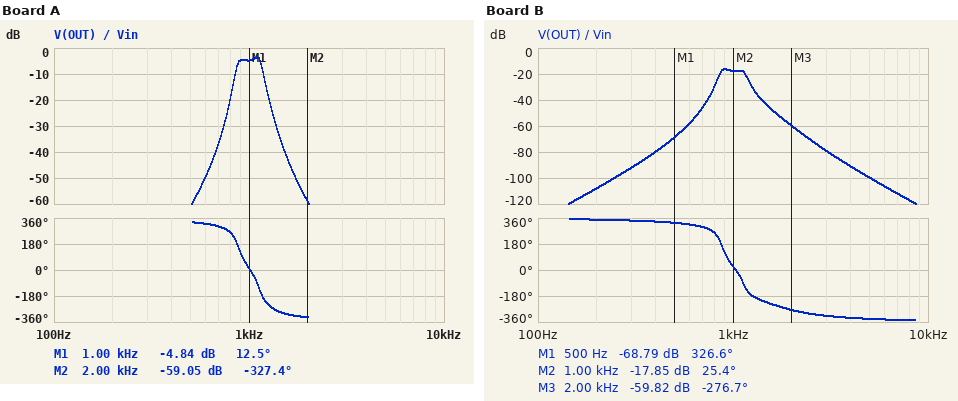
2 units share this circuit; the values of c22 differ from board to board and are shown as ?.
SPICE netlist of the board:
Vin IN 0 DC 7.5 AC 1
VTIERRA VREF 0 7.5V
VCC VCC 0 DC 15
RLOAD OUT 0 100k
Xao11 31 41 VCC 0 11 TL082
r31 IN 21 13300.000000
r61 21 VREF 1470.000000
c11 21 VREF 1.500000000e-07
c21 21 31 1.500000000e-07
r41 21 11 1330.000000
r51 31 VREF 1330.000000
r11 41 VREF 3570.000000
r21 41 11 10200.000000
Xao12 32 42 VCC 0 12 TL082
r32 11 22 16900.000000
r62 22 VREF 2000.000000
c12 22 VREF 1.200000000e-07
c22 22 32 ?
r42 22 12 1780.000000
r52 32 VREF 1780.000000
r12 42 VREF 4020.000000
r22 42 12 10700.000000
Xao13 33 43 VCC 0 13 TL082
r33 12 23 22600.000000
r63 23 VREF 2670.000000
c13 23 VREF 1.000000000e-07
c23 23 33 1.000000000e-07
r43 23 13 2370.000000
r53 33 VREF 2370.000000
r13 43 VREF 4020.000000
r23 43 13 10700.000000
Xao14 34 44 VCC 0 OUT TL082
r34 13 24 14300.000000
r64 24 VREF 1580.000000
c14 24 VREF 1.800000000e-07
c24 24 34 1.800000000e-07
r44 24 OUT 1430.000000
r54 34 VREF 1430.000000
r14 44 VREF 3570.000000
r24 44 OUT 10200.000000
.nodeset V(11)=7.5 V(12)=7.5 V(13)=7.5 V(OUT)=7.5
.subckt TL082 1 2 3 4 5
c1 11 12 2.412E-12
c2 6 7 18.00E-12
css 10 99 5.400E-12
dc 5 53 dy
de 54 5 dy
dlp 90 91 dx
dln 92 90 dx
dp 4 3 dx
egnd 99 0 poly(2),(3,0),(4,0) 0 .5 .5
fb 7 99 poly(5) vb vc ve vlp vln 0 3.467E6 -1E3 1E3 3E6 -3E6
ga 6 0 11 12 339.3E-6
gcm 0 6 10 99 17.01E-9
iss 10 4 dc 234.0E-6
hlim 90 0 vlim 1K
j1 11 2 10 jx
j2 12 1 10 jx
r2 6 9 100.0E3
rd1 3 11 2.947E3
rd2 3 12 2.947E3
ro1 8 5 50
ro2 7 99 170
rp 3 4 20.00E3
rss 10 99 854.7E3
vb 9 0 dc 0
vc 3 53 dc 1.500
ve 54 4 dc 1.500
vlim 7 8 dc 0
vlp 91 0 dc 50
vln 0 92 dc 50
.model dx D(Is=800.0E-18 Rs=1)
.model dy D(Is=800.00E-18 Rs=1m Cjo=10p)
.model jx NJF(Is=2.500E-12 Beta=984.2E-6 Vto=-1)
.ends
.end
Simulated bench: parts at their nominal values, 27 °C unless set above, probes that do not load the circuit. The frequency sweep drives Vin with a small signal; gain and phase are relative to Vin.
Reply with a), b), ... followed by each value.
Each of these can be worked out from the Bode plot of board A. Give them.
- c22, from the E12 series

a) 100 nF
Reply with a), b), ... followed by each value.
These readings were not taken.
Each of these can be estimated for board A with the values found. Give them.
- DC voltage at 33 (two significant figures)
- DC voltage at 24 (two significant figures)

a) 7.5 V
b) 7.5 V
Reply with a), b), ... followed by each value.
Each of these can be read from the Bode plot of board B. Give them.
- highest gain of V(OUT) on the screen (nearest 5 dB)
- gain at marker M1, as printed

a) -15 dB
b) -68.79 dB
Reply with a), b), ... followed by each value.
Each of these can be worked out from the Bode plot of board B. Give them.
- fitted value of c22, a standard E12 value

a) 47 nF
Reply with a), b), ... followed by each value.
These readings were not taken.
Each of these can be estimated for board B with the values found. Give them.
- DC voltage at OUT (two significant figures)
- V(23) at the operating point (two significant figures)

a) 7.5 V
b) 7.5 V
